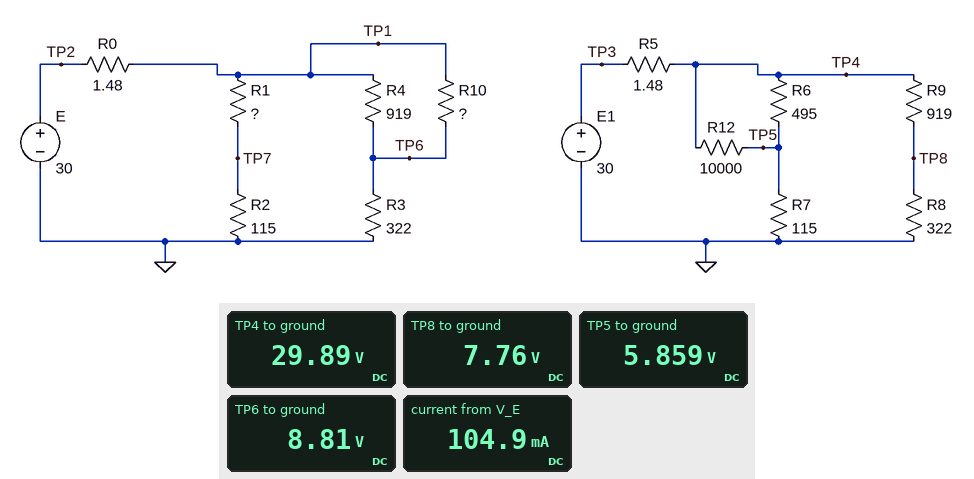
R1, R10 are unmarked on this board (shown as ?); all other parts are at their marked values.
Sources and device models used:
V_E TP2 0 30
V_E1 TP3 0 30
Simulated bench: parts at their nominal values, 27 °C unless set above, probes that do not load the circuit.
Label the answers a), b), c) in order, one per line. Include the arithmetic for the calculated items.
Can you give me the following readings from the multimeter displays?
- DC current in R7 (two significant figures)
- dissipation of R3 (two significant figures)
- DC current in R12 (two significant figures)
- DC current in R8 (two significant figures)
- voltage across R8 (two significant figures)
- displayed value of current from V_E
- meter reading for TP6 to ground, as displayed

a) (5.859 V) / 115 Ω = 51 mA
b) (8.81 V)^2 / 322 Ω = 240 mW
c) (29.89 V - 5.859 V) / 10 kΩ = 2.4 mA
d) (7.76 V) / 322 Ω = 24 mA
e) 7.76 V = 7.8 V
f) 104.9 mA
g) 8.81 V
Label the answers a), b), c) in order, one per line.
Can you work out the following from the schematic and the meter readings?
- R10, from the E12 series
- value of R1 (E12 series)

a) 4.7 kΩ
b) 270 Ω
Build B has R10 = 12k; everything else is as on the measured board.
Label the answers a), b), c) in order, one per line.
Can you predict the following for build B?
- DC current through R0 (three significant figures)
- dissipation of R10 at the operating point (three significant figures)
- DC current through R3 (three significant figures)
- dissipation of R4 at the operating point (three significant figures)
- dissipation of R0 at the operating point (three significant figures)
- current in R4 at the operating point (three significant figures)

a) 103 mA
b) 39.1 mW
c) 25.4 mA
d) 511 mW
e) 15.7 mW
f) 23.6 mA
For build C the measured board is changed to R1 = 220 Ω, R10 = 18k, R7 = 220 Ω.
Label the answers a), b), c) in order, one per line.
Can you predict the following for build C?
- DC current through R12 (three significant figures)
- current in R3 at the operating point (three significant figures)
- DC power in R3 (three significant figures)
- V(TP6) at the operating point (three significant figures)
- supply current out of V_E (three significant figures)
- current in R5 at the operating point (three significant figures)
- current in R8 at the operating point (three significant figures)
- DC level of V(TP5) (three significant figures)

a) 2.04 mA
b) 24.9 mA
c) 200 mW
d) 8.03 V
e) 114 mA
f) 67.3 mA
g) 24.1 mA
h) 9.51 V
